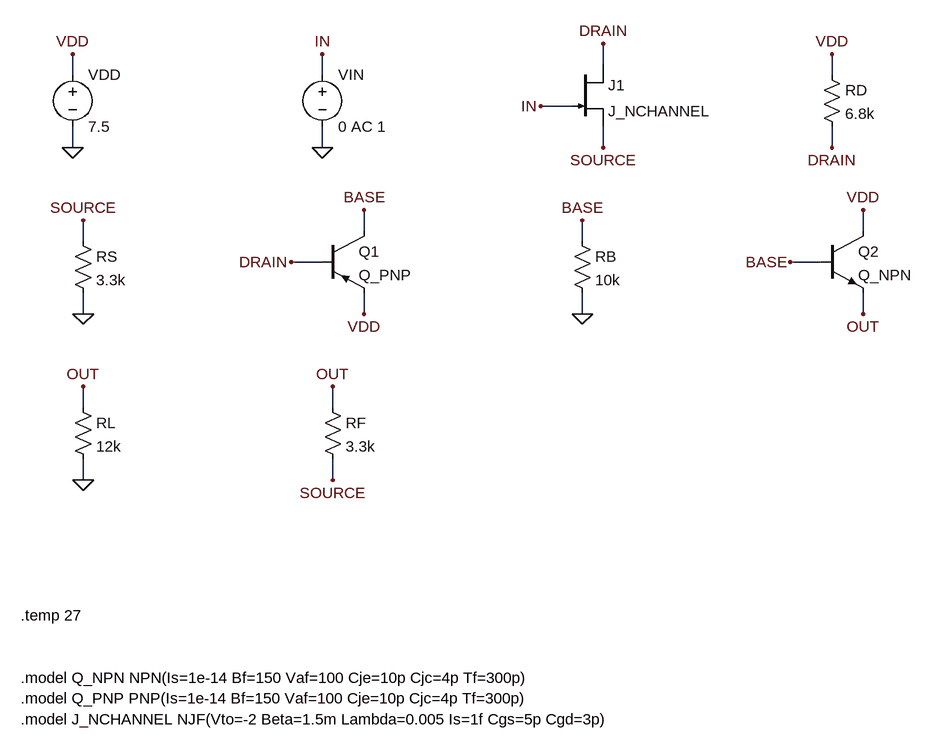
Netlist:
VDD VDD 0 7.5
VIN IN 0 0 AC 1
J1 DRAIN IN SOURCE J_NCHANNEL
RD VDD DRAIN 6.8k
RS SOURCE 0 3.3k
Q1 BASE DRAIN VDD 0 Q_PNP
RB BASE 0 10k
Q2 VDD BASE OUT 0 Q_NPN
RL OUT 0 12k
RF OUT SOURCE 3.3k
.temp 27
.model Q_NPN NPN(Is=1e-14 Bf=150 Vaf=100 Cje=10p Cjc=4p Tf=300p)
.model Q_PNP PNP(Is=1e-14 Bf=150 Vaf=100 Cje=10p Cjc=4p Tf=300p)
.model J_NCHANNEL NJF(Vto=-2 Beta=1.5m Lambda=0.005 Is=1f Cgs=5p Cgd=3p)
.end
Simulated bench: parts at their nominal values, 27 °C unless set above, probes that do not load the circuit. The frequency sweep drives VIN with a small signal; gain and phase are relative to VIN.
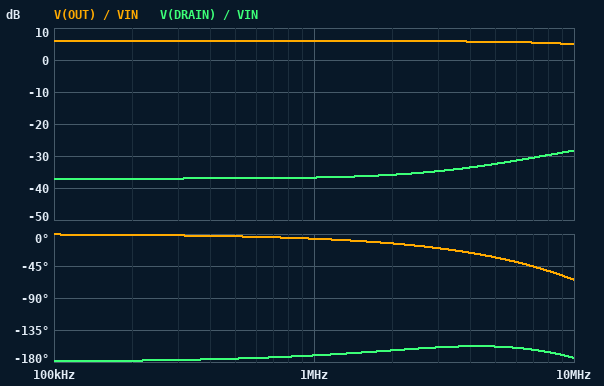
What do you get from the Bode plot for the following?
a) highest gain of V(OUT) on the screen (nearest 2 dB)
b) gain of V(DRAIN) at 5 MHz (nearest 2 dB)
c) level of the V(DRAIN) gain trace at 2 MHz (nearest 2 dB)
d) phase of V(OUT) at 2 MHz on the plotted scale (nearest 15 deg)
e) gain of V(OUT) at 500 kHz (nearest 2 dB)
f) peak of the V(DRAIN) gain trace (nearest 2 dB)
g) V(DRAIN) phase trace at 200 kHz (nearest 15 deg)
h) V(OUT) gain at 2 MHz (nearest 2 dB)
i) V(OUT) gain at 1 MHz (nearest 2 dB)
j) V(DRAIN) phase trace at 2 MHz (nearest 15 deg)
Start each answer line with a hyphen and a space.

- 6 dB
- -32 dB
- -36 dB
- -15 deg
- 6 dB
- -28 dB
- -180 deg
- 6 dB
- 6 dB
- -165 deg
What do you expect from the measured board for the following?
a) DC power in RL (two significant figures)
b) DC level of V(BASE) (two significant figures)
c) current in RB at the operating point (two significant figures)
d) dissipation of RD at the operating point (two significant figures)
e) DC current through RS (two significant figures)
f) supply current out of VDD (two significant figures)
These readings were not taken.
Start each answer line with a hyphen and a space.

- 850 µW
- 3.8 V
- 380 µA
- 58 µW
- 530 µA
- 1.2 mA
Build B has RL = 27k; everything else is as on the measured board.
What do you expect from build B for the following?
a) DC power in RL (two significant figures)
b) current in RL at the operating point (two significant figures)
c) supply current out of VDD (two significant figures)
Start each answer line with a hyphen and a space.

- 380 µW
- 120 µA
- 1.0 mA
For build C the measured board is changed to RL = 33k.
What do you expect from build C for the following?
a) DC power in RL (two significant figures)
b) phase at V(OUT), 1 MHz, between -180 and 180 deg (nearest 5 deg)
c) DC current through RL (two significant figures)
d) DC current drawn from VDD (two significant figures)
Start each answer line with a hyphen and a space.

- 310 µW
- -5 deg
- 97 µA
- 1.0 mA
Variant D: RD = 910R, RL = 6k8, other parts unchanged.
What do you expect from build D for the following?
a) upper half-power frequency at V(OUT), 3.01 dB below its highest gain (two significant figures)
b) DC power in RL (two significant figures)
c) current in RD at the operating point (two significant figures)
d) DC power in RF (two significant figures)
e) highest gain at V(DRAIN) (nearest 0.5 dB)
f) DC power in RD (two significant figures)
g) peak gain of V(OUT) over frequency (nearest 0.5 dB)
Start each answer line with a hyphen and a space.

- 16 MHz
- 130 µW
- 560 µA
- 63 µW
- -10.5 dB
- 290 µW
- -5.0 dB
